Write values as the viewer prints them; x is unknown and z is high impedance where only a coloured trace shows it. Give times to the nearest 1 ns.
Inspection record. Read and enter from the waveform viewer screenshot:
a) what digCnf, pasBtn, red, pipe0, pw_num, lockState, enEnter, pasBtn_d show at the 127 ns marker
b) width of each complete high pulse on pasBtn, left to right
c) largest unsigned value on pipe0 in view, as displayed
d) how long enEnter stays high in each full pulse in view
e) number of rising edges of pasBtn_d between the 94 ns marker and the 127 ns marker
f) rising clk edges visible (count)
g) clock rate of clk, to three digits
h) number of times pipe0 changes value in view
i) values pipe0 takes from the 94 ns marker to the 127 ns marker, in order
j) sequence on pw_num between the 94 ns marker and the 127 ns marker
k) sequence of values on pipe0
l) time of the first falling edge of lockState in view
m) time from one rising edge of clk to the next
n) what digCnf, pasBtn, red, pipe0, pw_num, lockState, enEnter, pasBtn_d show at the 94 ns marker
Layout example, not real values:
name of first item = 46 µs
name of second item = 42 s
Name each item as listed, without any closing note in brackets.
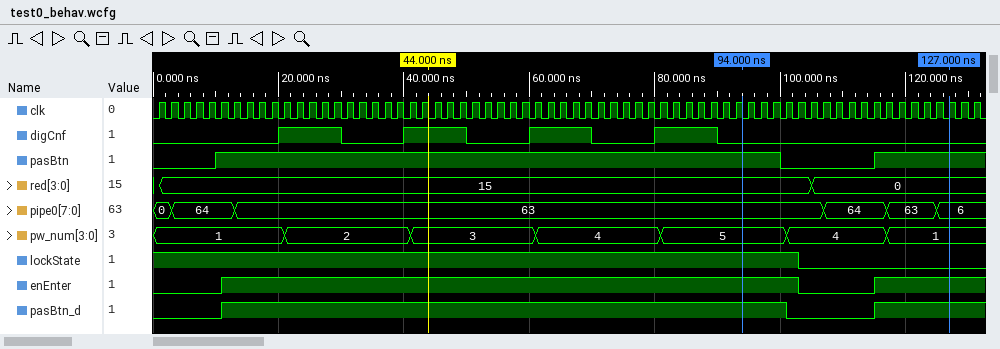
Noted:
what digCnf, pasBtn, red, pipe0, pw_num, lockState, enEnter, pasBtn_d show at the 127 ns marker = digCnf=0, pasBtn=1, red=0, pipe0=6, pw_num=1, lockState=0, enEnter=1, pasBtn_d=1
width of each complete high pulse on pasBtn, left to right = 90 ns
largest unsigned value on pipe0 in view, as displayed = 64
how long enEnter stays high in each full pulse in view = 92 ns
number of rising edges of pasBtn_d between the 94 ns marker and the 127 ns marker = 1
rising clk edges visible = 66
clock rate of clk, to three digits = 500 MHz
number of times pipe0 changes value in view = 5
values pipe0 takes from the 94 ns marker to the 127 ns marker, in order = 63, 64, 63, 6
sequence on pw_num between the 94 ns marker and the 127 ns marker = 5, 4, 1
sequence of values on pipe0 = 0, 64, 63, 64, 63, 6
time of the first falling edge of lockState in view = 103 ns
time from one rising edge of clk to the next = 2 ns
what digCnf, pasBtn, red, pipe0, pw_num, lockState, enEnter, pasBtn_d show at the 94 ns marker = digCnf=0, pasBtn=1, red=15, pipe0=63, pw_num=5, lockState=1, enEnter=1, pasBtn_d=1
